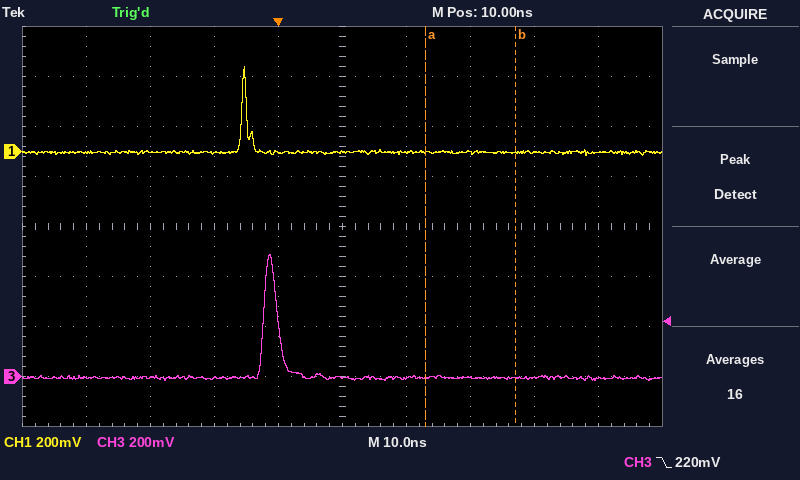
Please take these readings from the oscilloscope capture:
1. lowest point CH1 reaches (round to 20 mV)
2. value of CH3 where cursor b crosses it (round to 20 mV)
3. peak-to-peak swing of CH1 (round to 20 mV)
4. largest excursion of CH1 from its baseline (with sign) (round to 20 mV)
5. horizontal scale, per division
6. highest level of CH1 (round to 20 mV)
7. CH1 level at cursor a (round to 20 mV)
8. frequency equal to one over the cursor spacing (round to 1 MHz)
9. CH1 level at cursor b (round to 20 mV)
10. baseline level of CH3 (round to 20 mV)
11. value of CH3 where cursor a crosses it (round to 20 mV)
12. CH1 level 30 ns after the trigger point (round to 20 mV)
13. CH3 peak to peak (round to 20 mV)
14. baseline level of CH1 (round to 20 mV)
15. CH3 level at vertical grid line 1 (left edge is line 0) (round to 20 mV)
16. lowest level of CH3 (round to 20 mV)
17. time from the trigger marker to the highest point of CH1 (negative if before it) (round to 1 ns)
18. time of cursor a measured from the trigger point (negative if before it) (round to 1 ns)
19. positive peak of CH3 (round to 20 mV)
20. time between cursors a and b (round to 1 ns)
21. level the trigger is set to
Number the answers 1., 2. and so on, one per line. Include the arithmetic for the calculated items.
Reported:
1. -20 mV
2. 0 mV
3. 340 mV − (-20 mV) = 360 mV
4. 340 mV − (0 mV) = +340 mV
5. 10 ns
6. 340 mV
7. 0 mV
8. 1 / 14 ns ≈ 71 MHz
9. 0 mV
10. 0 mV
11. 0 mV
12. 0 mV
13. 480 mV − (-20 mV) = 500 mV
14. 0 mV
15. 0 mV
16. -20 mV
17. -5 ns
18. +23 ns
19. 480 mV
20. 14 ns
21. 220 mV
